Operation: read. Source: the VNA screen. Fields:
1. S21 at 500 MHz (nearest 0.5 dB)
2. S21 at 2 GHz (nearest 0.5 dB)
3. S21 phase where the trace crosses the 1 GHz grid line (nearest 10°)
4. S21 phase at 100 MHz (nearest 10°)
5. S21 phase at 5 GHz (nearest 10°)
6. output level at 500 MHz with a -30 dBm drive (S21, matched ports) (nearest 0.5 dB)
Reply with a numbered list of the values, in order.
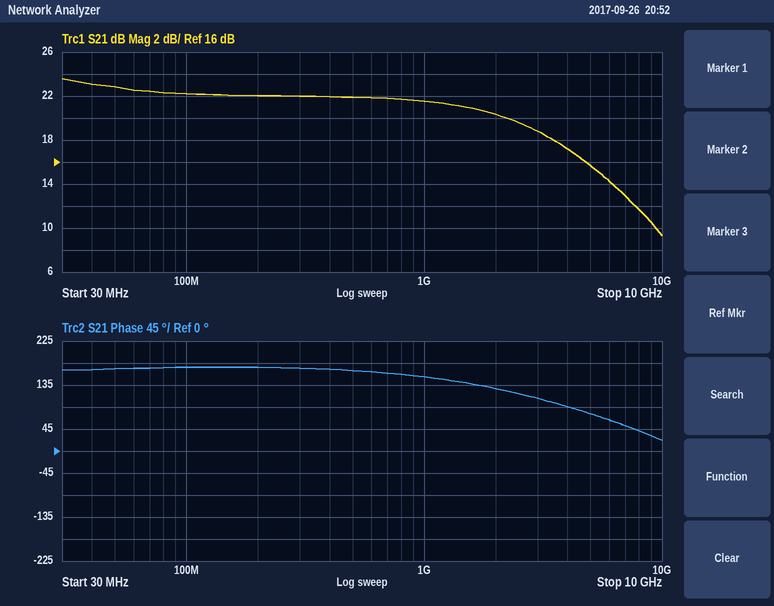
1. 22.0 dB
2. 20.5 dB
3. 150°
4. 170°
5. 80°
6. -8.0 dBm
